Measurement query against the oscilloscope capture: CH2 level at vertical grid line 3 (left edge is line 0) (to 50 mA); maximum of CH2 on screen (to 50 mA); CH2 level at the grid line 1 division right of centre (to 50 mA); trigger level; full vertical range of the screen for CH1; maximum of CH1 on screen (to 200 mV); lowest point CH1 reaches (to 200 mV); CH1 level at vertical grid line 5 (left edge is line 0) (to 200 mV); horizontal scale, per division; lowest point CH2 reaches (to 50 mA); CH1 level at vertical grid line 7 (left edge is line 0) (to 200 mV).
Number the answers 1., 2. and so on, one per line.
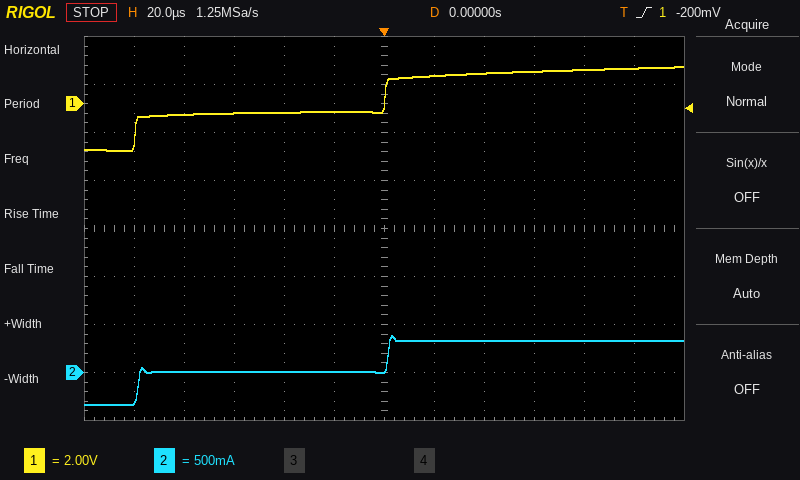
1. 0 mA
2. 400 mA
3. 350 mA
4. -200 mV
5. 16 V
6. 1.6 V
7. -2.0 V
8. -400 mV
9. 20 µs
10. -350 mA
11. 1.2 V
